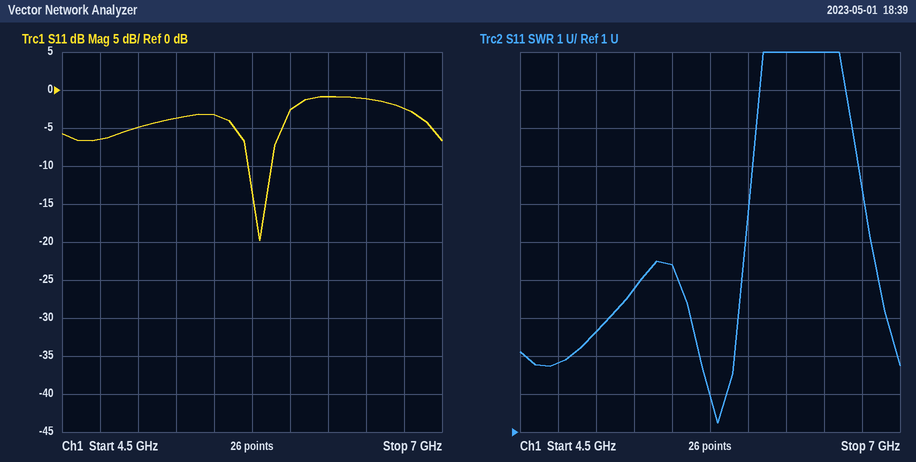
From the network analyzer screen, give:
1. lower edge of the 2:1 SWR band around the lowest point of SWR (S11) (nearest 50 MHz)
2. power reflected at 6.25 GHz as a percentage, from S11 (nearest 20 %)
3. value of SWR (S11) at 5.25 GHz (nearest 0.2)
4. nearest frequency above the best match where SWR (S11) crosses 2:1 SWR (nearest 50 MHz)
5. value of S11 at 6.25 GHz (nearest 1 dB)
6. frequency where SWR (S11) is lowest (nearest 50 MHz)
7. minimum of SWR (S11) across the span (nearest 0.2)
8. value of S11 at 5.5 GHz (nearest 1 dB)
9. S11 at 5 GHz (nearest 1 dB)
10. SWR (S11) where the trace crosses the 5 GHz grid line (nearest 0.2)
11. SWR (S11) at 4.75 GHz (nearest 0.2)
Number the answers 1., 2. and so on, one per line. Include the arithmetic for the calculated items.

1. 5.75 GHz
2. 10^(-1/10) ≈ 79.4 %, so 80 % to the nearest 20 %
3. 4.8
4. 5.85 GHz
5. -1 dB
6. 5.80 GHz
7. 1.2
8. -3 dB
9. -5 dB
10. 3.6
11. 2.8
